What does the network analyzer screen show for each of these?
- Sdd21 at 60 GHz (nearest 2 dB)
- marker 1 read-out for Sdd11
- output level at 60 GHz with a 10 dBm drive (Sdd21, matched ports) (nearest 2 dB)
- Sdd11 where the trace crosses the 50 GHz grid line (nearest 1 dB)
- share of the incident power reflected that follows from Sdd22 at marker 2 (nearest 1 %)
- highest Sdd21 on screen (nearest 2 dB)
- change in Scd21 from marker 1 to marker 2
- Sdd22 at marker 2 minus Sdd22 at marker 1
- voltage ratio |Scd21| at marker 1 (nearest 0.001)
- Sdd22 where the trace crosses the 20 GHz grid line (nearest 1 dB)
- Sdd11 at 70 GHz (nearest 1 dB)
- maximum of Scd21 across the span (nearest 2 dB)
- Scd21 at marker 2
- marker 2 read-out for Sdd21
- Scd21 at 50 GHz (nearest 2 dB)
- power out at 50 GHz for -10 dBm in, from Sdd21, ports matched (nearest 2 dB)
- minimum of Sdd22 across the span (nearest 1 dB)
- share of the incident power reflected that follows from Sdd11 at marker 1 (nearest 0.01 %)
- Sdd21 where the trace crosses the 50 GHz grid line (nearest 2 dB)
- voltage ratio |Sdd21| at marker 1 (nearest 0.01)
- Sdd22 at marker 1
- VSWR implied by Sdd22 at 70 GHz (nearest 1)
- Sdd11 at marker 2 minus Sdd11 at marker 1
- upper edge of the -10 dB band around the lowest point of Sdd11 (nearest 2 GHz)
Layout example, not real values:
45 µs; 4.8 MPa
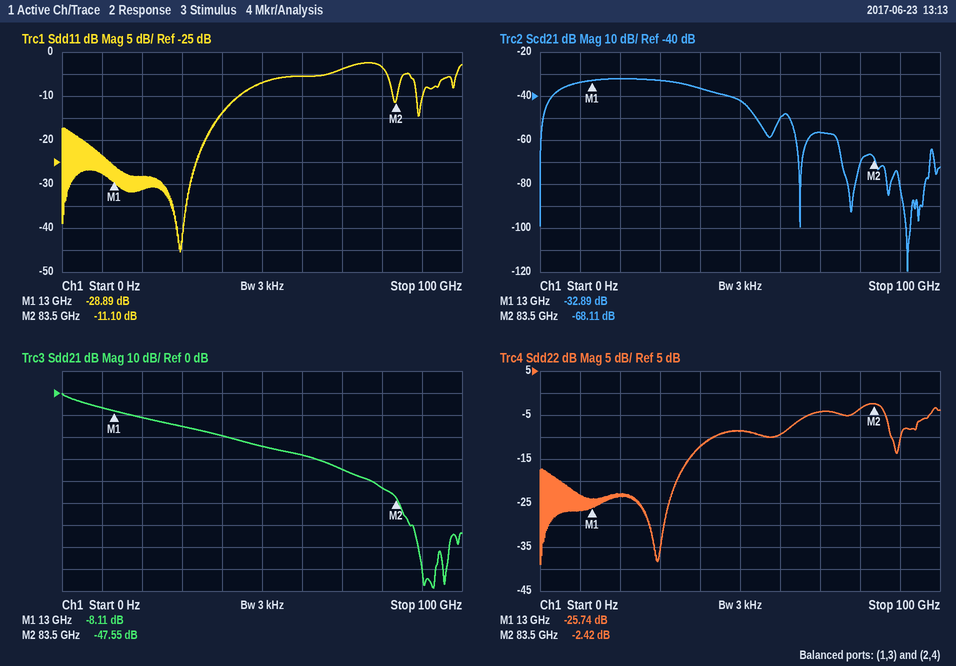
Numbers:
-28 dB; -28.89 dB; -18 dBm; -7 dB; 57 %; 0 dB; -35.22 dB; 23.32 dB; 0.023; -23 dB; -4 dB; -32 dB; -68.11 dB; -47.55 dB; -42 dB; -34 dBm; -39 dB; 0.13 %; -24 dB; 0.39; -25.74 dB; 4; 17.79 dB; 44 GHz
